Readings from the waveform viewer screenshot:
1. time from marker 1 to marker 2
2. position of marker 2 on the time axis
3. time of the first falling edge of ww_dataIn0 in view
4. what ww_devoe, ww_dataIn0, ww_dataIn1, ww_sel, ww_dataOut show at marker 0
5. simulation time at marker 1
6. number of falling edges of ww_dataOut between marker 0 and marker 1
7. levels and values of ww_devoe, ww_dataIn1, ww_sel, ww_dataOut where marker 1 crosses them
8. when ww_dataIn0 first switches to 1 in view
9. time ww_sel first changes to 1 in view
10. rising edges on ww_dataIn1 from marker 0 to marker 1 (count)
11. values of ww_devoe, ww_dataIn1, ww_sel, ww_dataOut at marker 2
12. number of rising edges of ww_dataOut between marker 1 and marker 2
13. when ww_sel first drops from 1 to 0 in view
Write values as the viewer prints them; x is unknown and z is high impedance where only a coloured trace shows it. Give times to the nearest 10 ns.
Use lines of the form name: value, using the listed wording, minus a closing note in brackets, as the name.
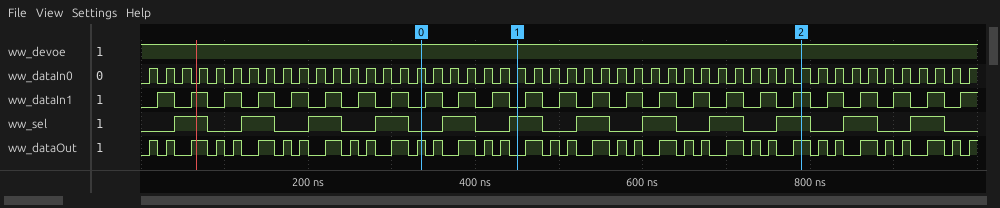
time from marker 1 to marker 2: 340 ns
position of marker 2 on the time axis: 790 ns
time of the first falling edge of ww_dataIn0 in view: 20 ns
what ww_devoe, ww_dataIn0, ww_dataIn1, ww_sel, ww_dataOut show at marker 0: ww_devoe=1, ww_dataIn0=1, ww_dataIn1=0, ww_sel=0, ww_dataOut=1
simulation time at marker 1: 450 ns
number of falling edges of ww_dataOut between marker 0 and marker 1: 5
levels and values of ww_devoe, ww_dataIn1, ww_sel, ww_dataOut where marker 1 crosses them: ww_devoe=1, ww_dataIn1=0, ww_sel=1, ww_dataOut=0
when ww_dataIn0 first switches to 1 in view: 10 ns
time ww_sel first changes to 1 in view: 40 ns
rising edges on ww_dataIn1 from marker 0 to marker 1: 3
values of ww_devoe, ww_dataIn1, ww_sel, ww_dataOut at marker 2: ww_devoe=1, ww_dataIn1=1, ww_sel=1, ww_dataOut=1
number of rising edges of ww_dataOut between marker 1 and marker 2: 13
when ww_sel first drops from 1 to 0 in view: 80 ns
